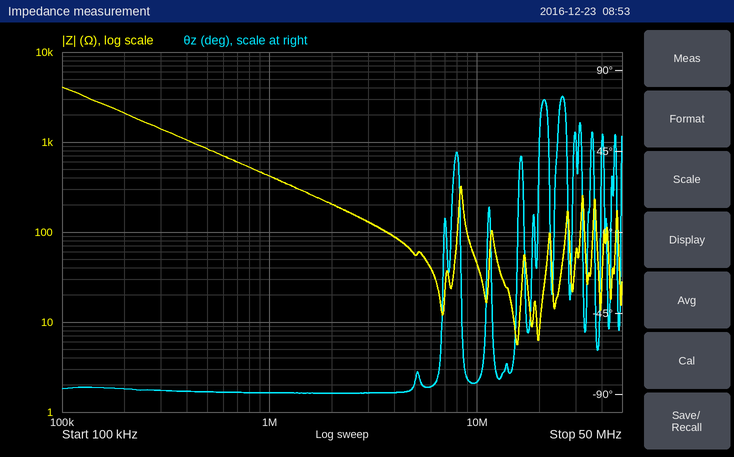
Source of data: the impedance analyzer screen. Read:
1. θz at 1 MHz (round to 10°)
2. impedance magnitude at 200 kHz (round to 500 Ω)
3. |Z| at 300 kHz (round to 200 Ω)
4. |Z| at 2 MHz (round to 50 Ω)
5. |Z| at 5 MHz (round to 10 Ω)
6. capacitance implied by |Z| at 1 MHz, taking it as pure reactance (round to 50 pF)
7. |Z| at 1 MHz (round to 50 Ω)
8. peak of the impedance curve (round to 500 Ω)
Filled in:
-90°
2.0 kΩ
1.4 kΩ
200 Ω
60 Ω
400 pF
400 Ω
4.0 kΩ
